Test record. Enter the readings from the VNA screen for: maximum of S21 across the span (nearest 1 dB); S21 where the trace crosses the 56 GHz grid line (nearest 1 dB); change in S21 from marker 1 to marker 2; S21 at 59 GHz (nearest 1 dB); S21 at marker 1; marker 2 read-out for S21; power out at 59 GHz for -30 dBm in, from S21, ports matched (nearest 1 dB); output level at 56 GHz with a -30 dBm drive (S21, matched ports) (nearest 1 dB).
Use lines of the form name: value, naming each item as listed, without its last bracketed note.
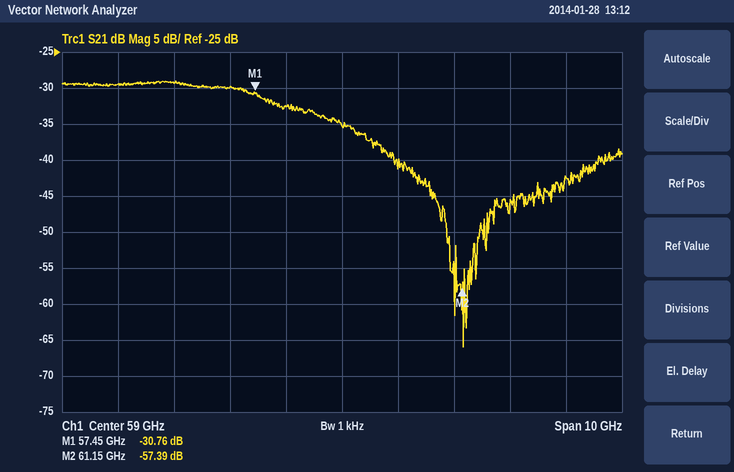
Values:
maximum of S21 across the span: -29 dB
S21 where the trace crosses the 56 GHz grid line: -29 dB
change in S21 from marker 1 to marker 2: -26.63 dB
S21 at 59 GHz: -35 dB
S21 at marker 1: -30.76 dB
marker 2 read-out for S21: -57.39 dB
power out at 59 GHz for -30 dBm in, from S21, ports matched: -65 dBm
output level at 56 GHz with a -30 dBm drive (S21, matched ports): -59 dBm
